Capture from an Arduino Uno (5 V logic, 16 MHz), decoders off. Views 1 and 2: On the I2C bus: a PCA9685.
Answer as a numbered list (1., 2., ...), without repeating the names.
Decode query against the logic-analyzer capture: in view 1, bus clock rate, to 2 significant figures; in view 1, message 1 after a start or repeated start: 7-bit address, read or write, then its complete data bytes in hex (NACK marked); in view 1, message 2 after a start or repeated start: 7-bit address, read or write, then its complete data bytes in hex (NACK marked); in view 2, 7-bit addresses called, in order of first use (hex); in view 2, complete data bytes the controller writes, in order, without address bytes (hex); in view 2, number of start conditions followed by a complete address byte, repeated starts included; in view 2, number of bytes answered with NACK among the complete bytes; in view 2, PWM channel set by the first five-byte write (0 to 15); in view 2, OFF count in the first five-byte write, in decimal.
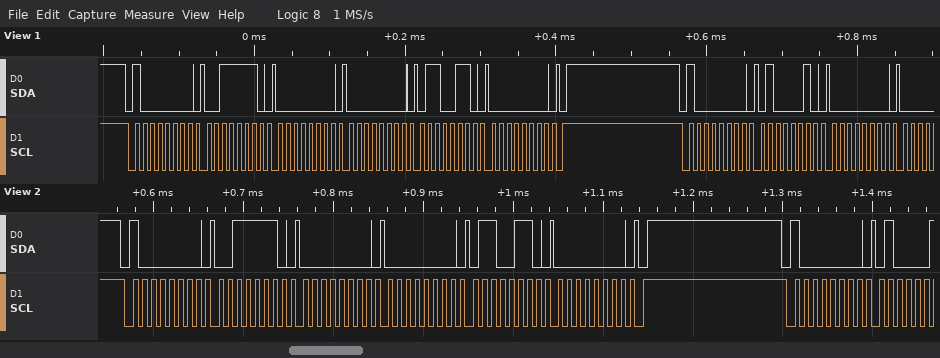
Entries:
1. 100 kHz
2. 0x40 write: 3E 00 00 66 00
3. 0x40 write: 42 00
4. 0x40
5. 3E 00 00 66 00
6. 2
7. 0
8. 14
9. 102
